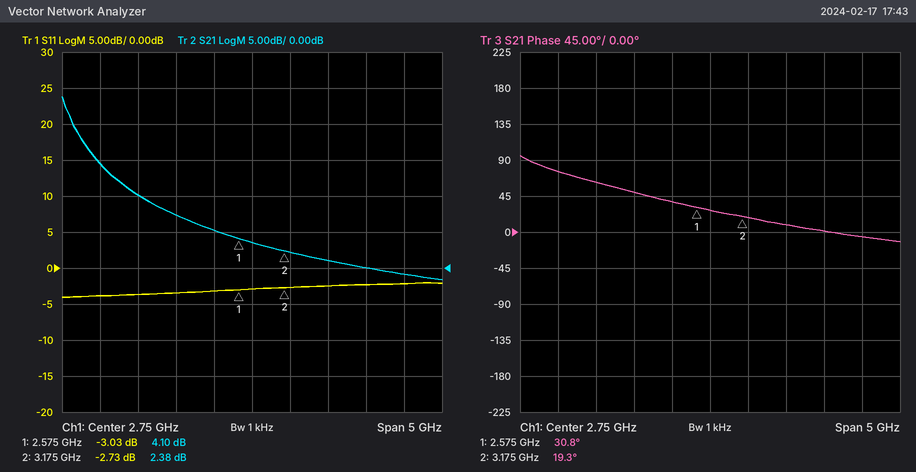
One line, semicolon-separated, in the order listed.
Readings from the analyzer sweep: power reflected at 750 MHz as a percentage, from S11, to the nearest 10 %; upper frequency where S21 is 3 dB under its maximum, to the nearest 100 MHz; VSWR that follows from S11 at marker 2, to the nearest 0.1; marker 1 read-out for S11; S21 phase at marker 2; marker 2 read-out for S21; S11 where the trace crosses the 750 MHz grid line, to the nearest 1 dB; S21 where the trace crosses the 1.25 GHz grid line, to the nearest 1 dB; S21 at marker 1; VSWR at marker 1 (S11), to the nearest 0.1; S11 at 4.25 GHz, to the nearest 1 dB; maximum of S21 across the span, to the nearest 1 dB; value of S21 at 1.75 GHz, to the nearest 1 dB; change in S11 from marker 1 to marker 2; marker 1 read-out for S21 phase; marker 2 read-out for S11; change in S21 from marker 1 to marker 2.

40 %; 400 MHz; 6.4; -3.03 dB; 19.3°; 2.38 dB; -4 dB; 10 dB; 4.10 dB; 5.8; -2 dB; 24 dB; 7 dB; 0.30 dB; 30.8°; -2.73 dB; -1.72 dB
